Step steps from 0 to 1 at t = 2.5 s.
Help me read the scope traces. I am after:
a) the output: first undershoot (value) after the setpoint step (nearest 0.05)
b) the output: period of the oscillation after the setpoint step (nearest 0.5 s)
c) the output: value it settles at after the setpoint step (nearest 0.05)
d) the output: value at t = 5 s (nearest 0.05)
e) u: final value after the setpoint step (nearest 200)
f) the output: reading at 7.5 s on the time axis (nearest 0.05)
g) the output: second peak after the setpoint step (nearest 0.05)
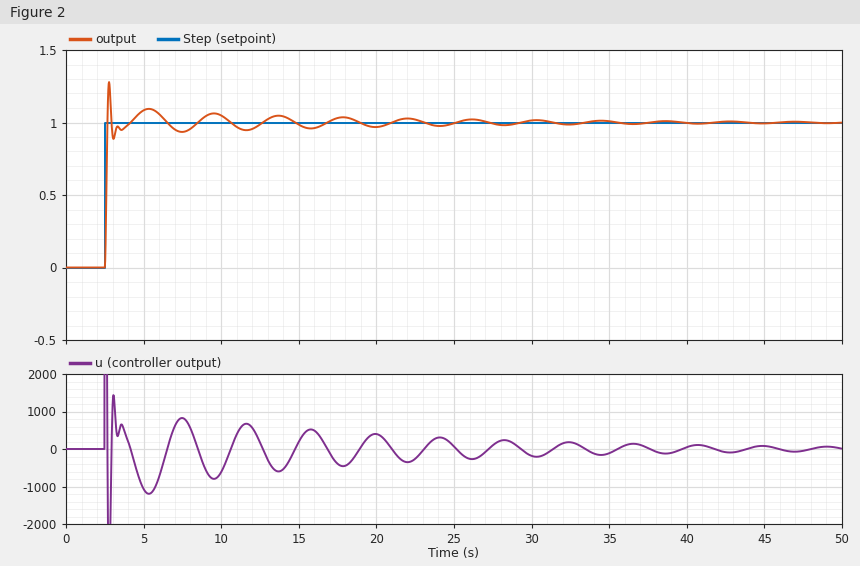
0.90
2.5 s
1.00
1.10
0
0.95
1.10
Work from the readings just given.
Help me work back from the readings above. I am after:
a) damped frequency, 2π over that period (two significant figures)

2.5 rad/s
